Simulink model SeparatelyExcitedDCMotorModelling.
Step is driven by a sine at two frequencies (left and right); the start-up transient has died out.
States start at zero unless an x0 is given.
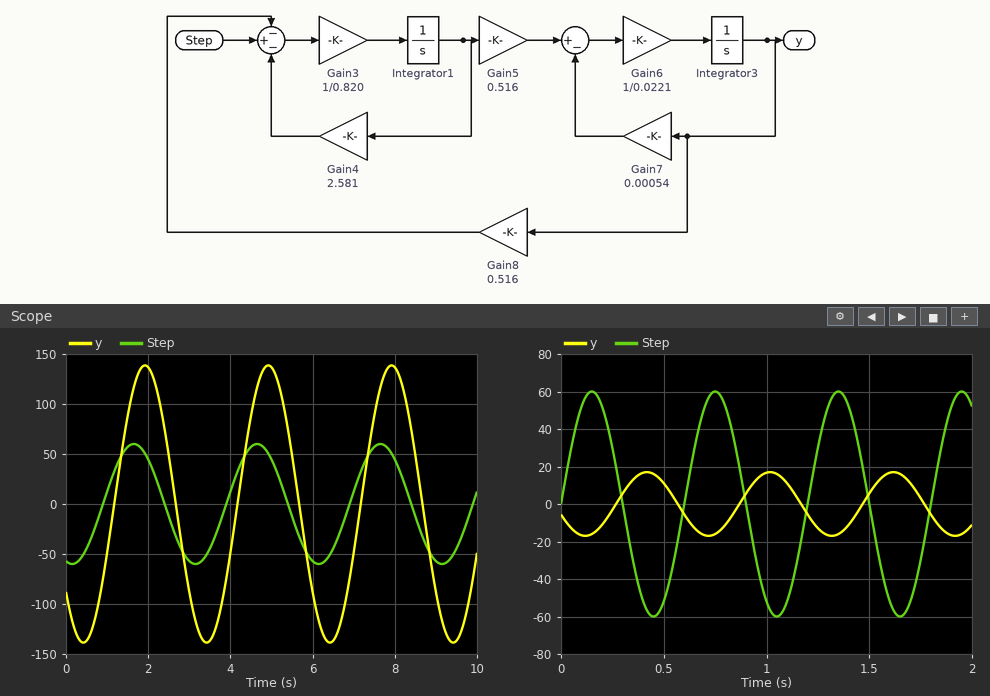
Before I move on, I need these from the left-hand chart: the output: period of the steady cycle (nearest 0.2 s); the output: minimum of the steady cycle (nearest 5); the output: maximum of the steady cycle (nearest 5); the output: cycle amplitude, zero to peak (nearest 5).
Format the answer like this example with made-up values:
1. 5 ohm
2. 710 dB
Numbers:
1. 3.0 s
2. -140
3. 140
4. 140
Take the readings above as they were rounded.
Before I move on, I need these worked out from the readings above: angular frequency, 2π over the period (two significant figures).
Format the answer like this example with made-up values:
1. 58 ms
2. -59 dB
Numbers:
1. 2.1 rad/s
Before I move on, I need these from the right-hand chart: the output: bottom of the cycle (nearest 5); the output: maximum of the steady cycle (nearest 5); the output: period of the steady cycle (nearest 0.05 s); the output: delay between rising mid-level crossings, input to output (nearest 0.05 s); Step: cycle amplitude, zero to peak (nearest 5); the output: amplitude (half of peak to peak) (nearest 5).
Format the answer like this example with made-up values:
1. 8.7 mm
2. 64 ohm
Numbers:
1. -15
2. 15
3. 0.60 s
4. 0.25 s
5. 60
6. 15
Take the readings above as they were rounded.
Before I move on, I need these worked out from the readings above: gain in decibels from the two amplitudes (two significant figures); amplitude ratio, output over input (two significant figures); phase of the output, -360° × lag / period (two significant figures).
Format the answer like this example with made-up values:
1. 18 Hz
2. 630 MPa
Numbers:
1. -12 dB
2. 0.25
3. -150°
